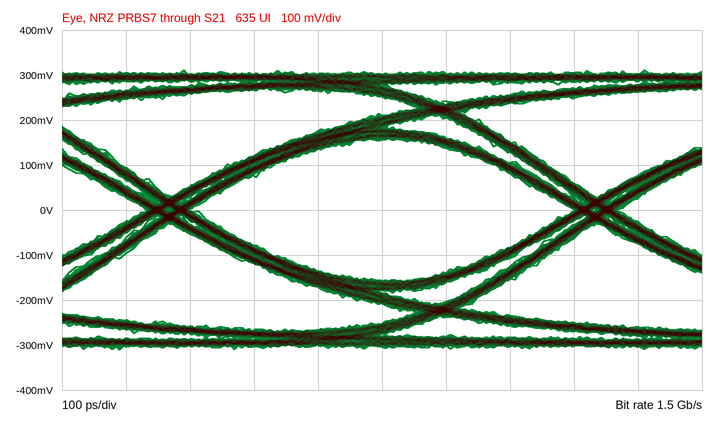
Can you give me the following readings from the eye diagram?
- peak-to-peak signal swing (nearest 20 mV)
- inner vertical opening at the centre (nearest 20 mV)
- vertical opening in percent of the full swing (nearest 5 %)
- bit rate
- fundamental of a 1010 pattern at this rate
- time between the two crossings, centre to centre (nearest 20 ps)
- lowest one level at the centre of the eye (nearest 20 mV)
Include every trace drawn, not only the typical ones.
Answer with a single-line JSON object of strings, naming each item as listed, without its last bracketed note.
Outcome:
{"peak-to-peak signal swing": "620 mV", "inner vertical opening at the centre": "320 mV", "vertical opening in percent of the full swing": "50 %", "bit rate": "1.5 Gb/s", "fundamental of a 1010 pattern at this rate": "750 MHz", "time between the two crossings, centre to centre": "660 ps", "lowest one level at the centre of the eye": "160 mV"}
